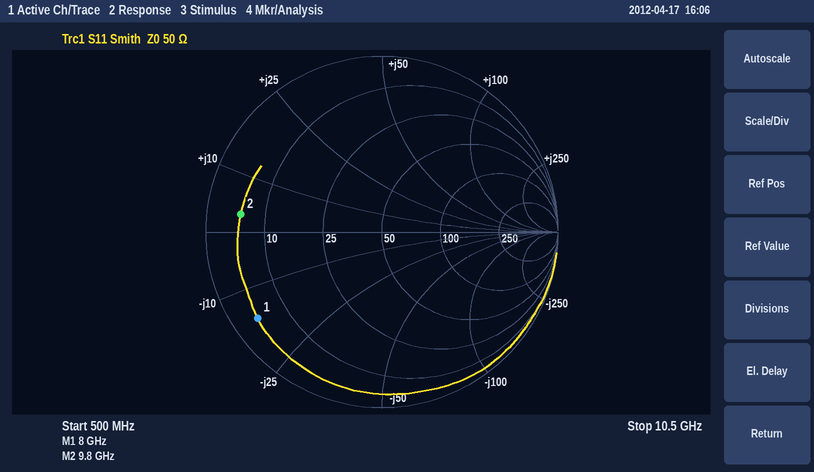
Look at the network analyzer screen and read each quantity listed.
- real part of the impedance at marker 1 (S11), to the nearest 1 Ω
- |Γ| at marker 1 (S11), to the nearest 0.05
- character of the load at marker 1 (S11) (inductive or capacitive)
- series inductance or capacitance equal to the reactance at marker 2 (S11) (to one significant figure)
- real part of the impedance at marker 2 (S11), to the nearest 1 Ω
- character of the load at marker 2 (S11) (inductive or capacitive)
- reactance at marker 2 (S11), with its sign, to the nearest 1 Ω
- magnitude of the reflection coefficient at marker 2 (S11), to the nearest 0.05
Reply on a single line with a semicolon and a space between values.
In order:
4 Ω; 0.85; capacitive; 50 pH; 5 Ω; inductive; +3 Ω; 0.80
